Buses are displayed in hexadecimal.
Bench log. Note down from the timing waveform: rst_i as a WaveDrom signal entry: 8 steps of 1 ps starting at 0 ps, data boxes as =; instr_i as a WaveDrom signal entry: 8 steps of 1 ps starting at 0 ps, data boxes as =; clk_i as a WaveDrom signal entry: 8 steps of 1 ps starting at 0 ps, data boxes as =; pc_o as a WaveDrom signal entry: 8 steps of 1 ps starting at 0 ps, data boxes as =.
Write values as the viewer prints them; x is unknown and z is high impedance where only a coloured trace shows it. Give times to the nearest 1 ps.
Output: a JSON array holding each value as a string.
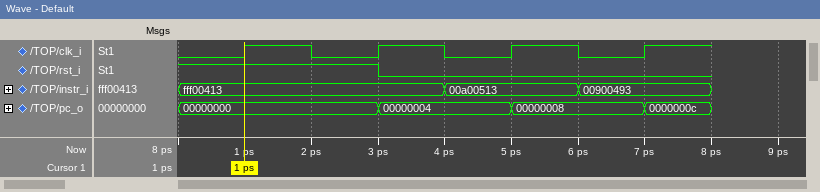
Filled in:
["{name: 'rst_i', wave: '1..0....'}", "{name: 'instr_i', wave: '=...=.=.', data: 'fff00413 00a00513 00900493'}", "{name: 'clk_i', wave: '01010101'}", "{name: 'pc_o', wave: '=..=.=.=', data: '00000000 00000004 00000008 0000000c'}"]
